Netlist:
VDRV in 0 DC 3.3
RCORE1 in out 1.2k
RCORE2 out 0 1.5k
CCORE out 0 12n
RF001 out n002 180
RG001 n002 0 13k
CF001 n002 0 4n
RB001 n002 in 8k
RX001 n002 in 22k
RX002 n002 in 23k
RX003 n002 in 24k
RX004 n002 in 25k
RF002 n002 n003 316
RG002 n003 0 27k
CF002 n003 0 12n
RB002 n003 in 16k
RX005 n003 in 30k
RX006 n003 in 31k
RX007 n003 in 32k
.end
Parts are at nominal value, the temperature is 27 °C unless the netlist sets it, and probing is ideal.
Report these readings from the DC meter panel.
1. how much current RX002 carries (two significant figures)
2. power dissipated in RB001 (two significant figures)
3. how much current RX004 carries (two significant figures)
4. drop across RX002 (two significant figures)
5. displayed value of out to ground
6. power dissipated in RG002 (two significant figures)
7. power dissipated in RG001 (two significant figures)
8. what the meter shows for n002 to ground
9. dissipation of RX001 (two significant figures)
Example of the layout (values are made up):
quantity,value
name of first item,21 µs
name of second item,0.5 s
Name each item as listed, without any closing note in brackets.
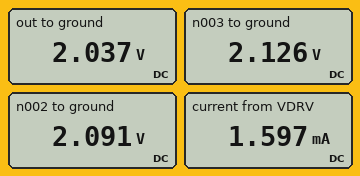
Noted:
quantity,value
how much current RX002 carries,53 µA
power dissipated in RB001,180 µW
how much current RX004 carries,48 µA
drop across RX002,1.2 V
displayed value of out to ground,2.037 V
power dissipated in RG002,170 µW
power dissipated in RG001,340 µW
what the meter shows for n002 to ground,2.091 V
dissipation of RX001,66 µW
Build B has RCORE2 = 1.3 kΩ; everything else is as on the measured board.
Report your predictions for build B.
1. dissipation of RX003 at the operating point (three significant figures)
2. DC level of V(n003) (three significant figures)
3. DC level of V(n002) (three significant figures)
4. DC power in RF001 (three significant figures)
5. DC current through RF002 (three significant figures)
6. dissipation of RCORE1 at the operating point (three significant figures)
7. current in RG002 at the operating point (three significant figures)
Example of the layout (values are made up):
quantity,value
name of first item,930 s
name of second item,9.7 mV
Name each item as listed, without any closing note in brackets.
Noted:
quantity,value
dissipation of RX003 at the operating point,70.3 µW
DC level of V(n003),2.04 V
DC level of V(n002),2.00 V
DC power in RF001,22.7 µW
DC current through RF002,125 µA
dissipation of RCORE1 at the operating point,1.55 mW
current in RG002 at the operating point,75.6 µA
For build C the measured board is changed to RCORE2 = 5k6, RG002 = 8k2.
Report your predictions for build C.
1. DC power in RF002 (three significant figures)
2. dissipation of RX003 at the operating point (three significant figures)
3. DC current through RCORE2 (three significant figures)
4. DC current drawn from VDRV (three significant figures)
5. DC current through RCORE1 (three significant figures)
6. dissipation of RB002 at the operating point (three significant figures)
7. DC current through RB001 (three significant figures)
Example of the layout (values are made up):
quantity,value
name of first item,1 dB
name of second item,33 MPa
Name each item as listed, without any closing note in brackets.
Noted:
quantity,value
DC power in RF002,9.64 µW
dissipation of RX003 at the operating point,23.7 µW
DC current through RCORE2,459 µA
DC current drawn from VDRV,959 µA
DC current through RCORE1,607 µA
dissipation of RB002 at the operating point,41.0 µW
DC current through RB001,94.3 µA
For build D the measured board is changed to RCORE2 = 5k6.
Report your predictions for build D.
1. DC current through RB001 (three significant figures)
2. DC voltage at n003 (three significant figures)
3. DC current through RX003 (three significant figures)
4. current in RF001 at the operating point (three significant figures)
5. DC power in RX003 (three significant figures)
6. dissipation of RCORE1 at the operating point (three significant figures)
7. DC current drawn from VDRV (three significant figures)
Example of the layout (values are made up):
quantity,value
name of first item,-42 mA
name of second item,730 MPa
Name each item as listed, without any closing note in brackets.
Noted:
quantity,value
DC current through RB001,76.7 µA
DC voltage at n003,2.69 V
DC current through RX003,25.6 µA
current in RF001 at the operating point,26.8 µA
DC power in RX003,15.7 µW
dissipation of RCORE1 at the operating point,309 µW
DC current drawn from VDRV,787 µA
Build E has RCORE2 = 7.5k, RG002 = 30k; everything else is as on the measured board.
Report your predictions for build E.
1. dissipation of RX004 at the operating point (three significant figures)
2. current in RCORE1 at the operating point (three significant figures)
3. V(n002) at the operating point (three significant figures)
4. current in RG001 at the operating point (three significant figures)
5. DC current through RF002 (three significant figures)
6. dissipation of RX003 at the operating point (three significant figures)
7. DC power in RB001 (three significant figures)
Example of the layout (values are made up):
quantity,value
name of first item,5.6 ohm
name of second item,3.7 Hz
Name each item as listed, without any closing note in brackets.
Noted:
quantity,value
dissipation of RX004 at the operating point,11.3 µW
current in RCORE1 at the operating point,434 µA
V(n002) at the operating point,2.77 V
current in RG001 at the operating point,213 µA
DC current through RF002,7.14 µA
dissipation of RX003 at the operating point,11.8 µW
DC power in RB001,35.3 µW
